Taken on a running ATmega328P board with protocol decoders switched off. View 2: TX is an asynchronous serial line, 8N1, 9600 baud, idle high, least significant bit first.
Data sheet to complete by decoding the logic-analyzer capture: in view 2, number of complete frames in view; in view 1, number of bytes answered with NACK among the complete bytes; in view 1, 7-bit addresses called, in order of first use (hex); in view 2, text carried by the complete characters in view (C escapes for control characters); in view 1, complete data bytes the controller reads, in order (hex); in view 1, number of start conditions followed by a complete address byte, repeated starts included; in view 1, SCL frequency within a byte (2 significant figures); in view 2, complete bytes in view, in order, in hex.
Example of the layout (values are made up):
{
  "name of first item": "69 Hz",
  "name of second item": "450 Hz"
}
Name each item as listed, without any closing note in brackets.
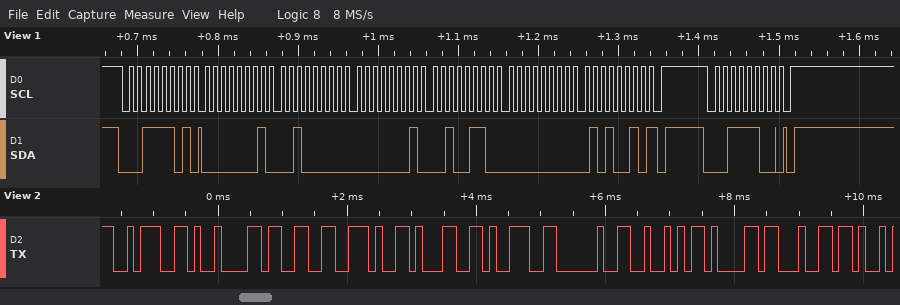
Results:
{
  "in view 2, number of complete frames in view": "10",
  "in view 1, number of bytes answered with NACK among the complete bytes": "1",
  "in view 1, 7-bit addresses called, in order of first use": "0x1E",
  "in view 2, text carried by the complete characters in view": "\":\\t3.19 Rad\"",
  "in view 1, complete data bytes the controller reads, in order": "01 20 01 26 00 52",
  "in view 1, number of start conditions followed by a complete address byte, repeated starts included": "2",
  "in view 1, SCL frequency within a byte": "100 kHz",
  "in view 2, complete bytes in view, in order, in hex": "3A 09 33 2E 31 39 20 52 61 64"
}
